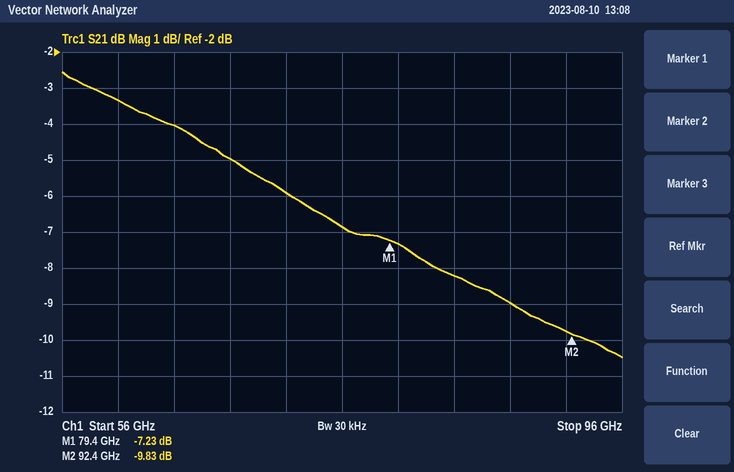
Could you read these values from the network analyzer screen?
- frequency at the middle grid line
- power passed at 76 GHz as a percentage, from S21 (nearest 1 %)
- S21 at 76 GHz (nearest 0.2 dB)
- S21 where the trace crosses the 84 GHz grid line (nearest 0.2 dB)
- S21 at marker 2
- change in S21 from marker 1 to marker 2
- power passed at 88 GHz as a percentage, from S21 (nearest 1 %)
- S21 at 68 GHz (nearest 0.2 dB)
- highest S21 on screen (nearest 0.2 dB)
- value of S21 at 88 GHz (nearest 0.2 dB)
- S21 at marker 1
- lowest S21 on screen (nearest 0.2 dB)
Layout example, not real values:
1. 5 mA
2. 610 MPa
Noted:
1. 76 GHz
2. 21 %
3. -6.8 dB
4. -8.2 dB
5. -9.83 dB
6. -2.60 dB
7. 13 %
8. -5.0 dB
9. -2.6 dB
10. -9.0 dB
11. -7.23 dB
12. -10.4 dB
